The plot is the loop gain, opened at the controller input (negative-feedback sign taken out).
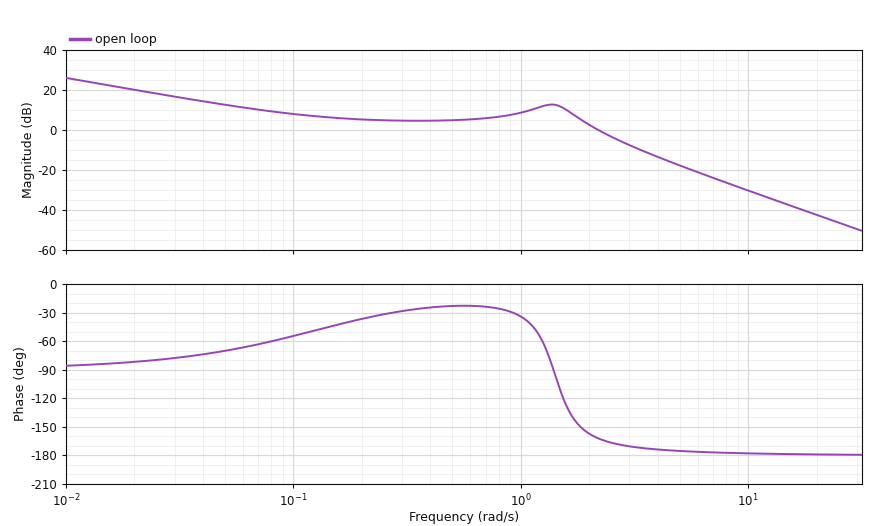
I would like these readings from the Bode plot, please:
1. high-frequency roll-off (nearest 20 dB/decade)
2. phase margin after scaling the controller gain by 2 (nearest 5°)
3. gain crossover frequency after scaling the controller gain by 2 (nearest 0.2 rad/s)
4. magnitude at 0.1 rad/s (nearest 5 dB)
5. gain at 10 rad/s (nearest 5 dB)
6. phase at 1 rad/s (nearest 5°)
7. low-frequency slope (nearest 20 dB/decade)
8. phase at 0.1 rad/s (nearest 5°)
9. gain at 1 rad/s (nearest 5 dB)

-40 dB/decade
10°
2.8 rad/s
10 dB
-30 dB
-35°
-20 dB/decade
-55°
10 dB
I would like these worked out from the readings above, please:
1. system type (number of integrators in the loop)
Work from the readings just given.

1
